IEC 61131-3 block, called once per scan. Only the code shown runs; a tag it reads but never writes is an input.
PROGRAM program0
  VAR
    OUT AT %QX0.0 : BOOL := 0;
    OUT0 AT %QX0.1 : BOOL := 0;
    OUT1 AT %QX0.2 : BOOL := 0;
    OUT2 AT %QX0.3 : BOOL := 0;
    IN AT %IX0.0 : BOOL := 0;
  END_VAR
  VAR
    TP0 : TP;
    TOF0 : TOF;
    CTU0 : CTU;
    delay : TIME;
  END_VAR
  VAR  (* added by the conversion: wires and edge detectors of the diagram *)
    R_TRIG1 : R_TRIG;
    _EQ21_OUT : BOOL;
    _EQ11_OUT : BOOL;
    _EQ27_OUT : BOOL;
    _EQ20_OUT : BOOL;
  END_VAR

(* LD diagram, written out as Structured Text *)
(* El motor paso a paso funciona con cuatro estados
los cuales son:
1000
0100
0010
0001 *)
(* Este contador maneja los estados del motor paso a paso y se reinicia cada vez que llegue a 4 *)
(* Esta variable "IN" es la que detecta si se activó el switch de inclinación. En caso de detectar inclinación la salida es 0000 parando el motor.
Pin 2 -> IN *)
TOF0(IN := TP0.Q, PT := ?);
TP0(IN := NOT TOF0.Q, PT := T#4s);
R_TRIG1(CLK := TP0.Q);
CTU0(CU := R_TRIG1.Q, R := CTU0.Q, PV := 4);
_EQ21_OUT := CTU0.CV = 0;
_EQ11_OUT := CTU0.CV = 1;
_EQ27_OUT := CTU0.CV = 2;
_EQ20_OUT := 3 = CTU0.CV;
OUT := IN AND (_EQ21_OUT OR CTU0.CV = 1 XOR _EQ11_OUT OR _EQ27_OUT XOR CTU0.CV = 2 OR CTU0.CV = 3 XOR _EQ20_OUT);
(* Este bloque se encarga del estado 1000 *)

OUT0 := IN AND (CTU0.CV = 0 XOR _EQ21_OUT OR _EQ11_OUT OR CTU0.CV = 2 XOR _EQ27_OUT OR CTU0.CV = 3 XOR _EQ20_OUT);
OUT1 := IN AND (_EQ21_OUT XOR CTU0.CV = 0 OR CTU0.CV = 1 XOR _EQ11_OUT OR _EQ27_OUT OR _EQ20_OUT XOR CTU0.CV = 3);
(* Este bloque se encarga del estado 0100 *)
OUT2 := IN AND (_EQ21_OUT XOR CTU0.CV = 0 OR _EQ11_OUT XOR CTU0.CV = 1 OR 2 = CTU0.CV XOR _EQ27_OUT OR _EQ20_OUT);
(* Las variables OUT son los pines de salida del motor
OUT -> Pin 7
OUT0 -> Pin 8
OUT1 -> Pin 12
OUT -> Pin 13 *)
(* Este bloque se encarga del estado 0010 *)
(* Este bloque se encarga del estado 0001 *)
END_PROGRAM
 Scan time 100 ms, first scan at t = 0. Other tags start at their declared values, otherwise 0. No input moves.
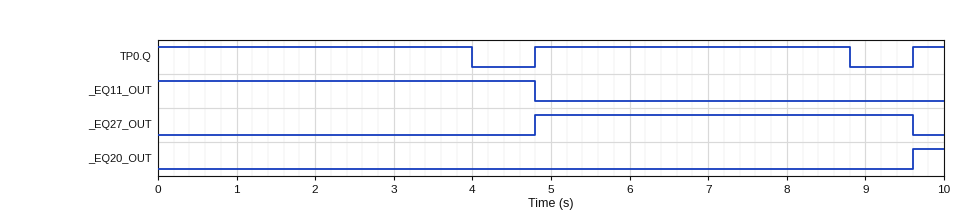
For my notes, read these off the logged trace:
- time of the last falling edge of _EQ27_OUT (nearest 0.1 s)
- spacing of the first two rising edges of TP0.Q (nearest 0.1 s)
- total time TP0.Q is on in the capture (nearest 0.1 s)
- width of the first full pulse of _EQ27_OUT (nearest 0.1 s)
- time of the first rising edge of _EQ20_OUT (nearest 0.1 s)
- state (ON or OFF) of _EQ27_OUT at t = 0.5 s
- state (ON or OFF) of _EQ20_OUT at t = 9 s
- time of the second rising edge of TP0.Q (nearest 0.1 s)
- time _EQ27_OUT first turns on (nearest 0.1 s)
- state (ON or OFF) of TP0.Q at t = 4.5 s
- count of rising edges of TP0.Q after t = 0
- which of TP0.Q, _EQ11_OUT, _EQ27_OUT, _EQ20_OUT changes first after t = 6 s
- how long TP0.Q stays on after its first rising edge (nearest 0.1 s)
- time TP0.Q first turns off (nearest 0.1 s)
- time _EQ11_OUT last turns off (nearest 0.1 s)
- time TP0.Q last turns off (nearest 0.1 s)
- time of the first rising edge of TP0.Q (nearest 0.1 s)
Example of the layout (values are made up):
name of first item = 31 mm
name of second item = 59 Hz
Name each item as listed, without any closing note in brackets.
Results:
time of the last falling edge of _EQ27_OUT = 9.6 s
spacing of the first two rising edges of TP0.Q = 4.8 s
total time TP0.Q is on in the capture = 8.4 s
width of the first full pulse of _EQ27_OUT = 4.8 s
time of the first rising edge of _EQ20_OUT = 9.6 s
state (ON or OFF) of _EQ27_OUT at t = 0.5 s = OFF
state (ON or OFF) of _EQ20_OUT at t = 9 s = OFF
time of the second rising edge of TP0.Q = 9.6 s
time _EQ27_OUT first turns on = 4.8 s
state (ON or OFF) of TP0.Q at t = 4.5 s = OFF
count of rising edges of TP0.Q after t = 0 = 2
which of TP0.Q, _EQ11_OUT, _EQ27_OUT, _EQ20_OUT changes first after t = 6 s = TP0.Q
how long TP0.Q stays on after its first rising edge = 4.0 s
time TP0.Q first turns off = 4.0 s
time _EQ11_OUT last turns off = 4.8 s
time TP0.Q last turns off = 8.8 s
time of the first rising edge of TP0.Q = 4.8 s
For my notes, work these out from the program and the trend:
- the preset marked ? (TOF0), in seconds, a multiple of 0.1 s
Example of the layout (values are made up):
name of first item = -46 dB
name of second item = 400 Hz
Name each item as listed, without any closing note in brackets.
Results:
the preset marked ? (TOF0), in seconds, a multiple of 0.1 s = 0.7 s
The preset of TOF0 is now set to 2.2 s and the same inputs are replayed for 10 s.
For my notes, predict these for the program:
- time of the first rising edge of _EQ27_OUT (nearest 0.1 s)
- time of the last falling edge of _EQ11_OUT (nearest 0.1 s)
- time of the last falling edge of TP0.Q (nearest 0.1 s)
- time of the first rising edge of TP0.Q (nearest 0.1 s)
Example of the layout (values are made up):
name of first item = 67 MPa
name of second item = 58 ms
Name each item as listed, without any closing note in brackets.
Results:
time of the first rising edge of _EQ27_OUT = 6.3 s
time of the last falling edge of _EQ11_OUT = 6.3 s
time of the last falling edge of TP0.Q = 4.0 s
time of the first rising edge of TP0.Q = 6.3 s
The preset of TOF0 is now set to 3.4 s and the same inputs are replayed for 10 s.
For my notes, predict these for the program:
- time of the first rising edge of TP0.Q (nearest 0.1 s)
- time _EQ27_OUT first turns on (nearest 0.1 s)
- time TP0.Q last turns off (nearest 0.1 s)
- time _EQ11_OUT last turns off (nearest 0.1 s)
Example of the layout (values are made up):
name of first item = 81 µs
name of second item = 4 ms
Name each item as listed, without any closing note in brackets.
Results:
time of the first rising edge of TP0.Q = 7.5 s
time _EQ27_OUT first turns on = 7.5 s
time TP0.Q last turns off = 4.0 s
time _EQ11_OUT last turns off = 7.5 s
